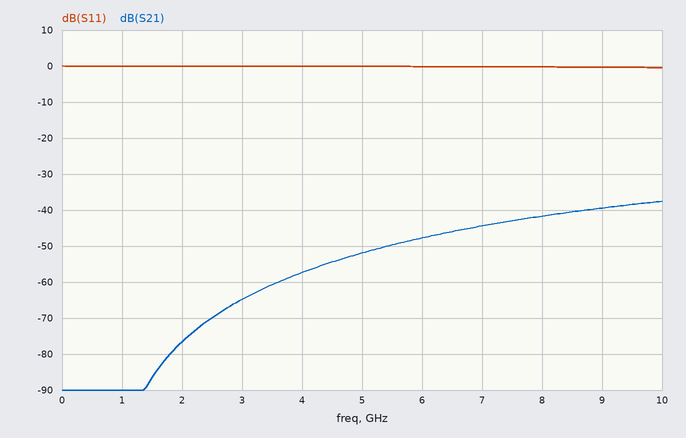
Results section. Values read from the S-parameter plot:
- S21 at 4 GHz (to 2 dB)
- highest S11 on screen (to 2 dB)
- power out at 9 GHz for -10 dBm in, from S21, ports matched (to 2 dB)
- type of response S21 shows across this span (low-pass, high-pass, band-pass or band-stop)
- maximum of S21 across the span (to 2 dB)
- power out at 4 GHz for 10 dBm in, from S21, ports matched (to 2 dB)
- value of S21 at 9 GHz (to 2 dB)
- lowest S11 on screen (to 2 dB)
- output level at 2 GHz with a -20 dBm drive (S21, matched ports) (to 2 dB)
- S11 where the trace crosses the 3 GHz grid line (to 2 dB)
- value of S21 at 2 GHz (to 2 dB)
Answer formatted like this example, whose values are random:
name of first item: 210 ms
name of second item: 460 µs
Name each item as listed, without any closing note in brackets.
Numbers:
S21 at 4 GHz: -58 dB
highest S11 on screen: 0 dB
power out at 9 GHz for -10 dBm in, from S21, ports matched: -50 dBm
type of response S21 shows across this span: high-pass
maximum of S21 across the span: -38 dB
power out at 4 GHz for 10 dBm in, from S21, ports matched: -48 dBm
value of S21 at 9 GHz: -40 dB
lowest S11 on screen: 0 dB
output level at 2 GHz with a -20 dBm drive (S21, matched ports): -96 dBm
S11 where the trace crosses the 3 GHz grid line: 0 dB
value of S21 at 2 GHz: -76 dB
